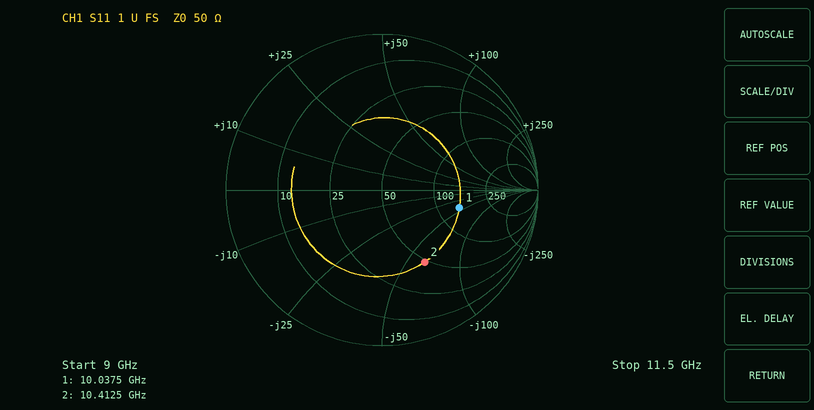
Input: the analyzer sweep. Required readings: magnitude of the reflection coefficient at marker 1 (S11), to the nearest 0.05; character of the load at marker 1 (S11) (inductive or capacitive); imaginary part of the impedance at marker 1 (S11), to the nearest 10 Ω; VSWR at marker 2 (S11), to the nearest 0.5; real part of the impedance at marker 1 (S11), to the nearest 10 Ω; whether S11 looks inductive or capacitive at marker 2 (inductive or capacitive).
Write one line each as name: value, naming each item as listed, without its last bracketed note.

magnitude of the reflection coefficient at marker 1 (S11), to the nearest 0.05: 0.50
character of the load at marker 1 (S11): capacitive
imaginary part of the impedance at marker 1 (S11), to the nearest 10 Ω: -40 Ω
VSWR at marker 2 (S11), to the nearest 0.5: 3.5
real part of the impedance at marker 1 (S11), to the nearest 10 Ω: 140 Ω
whether S11 looks inductive or capacitive at marker 2: capacitive
